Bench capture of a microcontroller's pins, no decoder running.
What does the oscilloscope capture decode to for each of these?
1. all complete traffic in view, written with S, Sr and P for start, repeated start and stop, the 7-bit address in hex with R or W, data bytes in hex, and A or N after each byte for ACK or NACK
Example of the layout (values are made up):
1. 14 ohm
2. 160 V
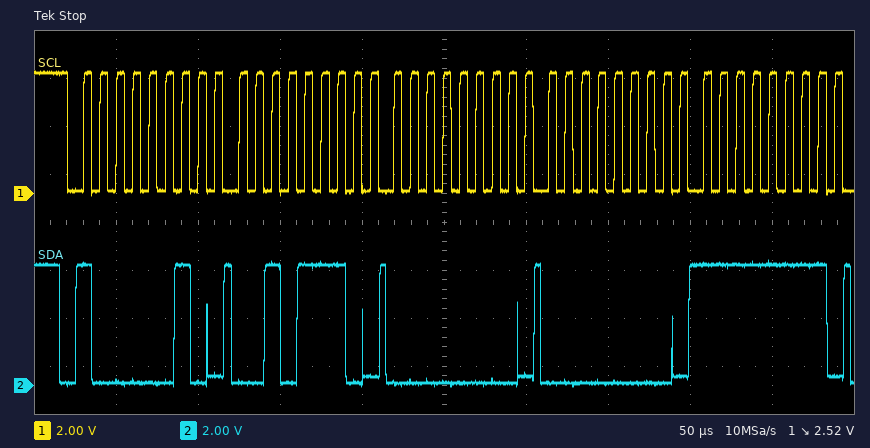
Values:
1. S 41W A 2E A 00 A 00 A FF A
